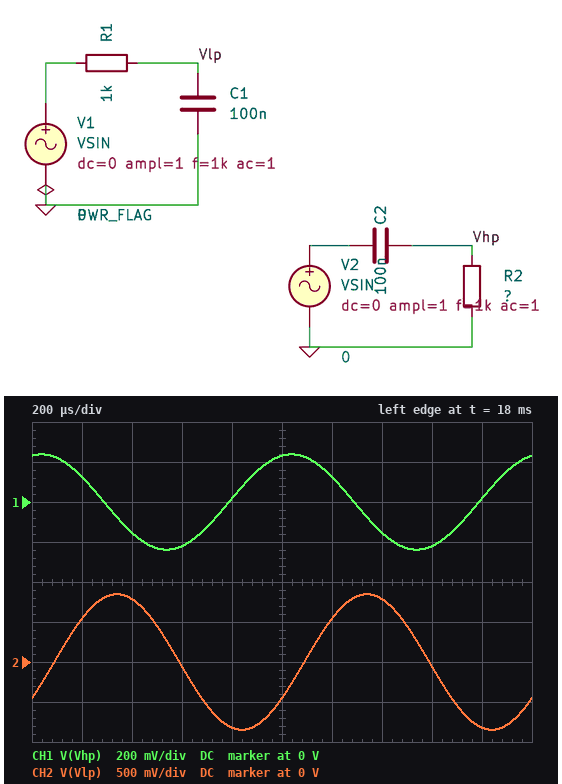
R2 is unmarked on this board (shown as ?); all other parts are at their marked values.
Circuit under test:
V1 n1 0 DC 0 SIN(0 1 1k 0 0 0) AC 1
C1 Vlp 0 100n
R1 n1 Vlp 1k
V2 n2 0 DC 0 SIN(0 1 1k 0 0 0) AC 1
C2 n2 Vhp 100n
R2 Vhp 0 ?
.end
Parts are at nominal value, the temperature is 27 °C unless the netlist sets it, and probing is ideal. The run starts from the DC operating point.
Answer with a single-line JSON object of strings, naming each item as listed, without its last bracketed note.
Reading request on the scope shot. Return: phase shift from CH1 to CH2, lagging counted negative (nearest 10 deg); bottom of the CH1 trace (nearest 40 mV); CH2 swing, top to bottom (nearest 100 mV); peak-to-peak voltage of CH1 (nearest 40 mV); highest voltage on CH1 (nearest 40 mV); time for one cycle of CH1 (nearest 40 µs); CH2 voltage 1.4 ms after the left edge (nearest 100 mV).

{"phase shift from CH1 to CH2, lagging counted negative": "-110 deg", "bottom of the CH1 trace": "-240 mV", "CH2 swing, top to bottom": "1.7 V", "peak-to-peak voltage of CH1": "480 mV", "highest voltage on CH1": "240 mV", "time for one cycle of CH1": "1.00 ms", "CH2 voltage 1.4 ms after the left edge": "800 mV"}
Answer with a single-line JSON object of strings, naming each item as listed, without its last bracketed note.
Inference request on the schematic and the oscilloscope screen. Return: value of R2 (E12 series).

{"value of R2": "390 Ω"}
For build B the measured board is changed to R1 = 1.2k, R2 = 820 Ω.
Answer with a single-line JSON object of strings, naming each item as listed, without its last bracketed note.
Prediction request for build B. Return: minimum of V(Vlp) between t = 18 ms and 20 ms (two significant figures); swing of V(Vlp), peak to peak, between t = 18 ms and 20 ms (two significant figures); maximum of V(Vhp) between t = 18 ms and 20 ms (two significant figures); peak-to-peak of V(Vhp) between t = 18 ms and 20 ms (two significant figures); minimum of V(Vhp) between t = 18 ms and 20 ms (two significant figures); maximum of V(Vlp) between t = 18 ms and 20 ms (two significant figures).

{"minimum of V(Vlp) between t = 18 ms and 20 ms": "-800 mV", "swing of V(Vlp), peak to peak, between t = 18 ms and 20 ms": "1.6 V", "maximum of V(Vhp) between t = 18 ms and 20 ms": "460 mV", "peak-to-peak of V(Vhp) between t = 18 ms and 20 ms": "920 mV", "minimum of V(Vhp) between t = 18 ms and 20 ms": "-460 mV", "maximum of V(Vlp) between t = 18 ms and 20 ms": "800 mV"}
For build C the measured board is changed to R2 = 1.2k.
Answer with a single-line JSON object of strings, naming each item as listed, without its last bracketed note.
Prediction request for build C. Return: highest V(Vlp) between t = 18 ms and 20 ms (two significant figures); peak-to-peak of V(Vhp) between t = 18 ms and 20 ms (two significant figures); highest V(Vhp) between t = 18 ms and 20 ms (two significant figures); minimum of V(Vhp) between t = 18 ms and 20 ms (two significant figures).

{"highest V(Vlp) between t = 18 ms and 20 ms": "850 mV", "peak-to-peak of V(Vhp) between t = 18 ms and 20 ms": "1.2 V", "highest V(Vhp) between t = 18 ms and 20 ms": "600 mV", "minimum of V(Vhp) between t = 18 ms and 20 ms": "-600 mV"}
